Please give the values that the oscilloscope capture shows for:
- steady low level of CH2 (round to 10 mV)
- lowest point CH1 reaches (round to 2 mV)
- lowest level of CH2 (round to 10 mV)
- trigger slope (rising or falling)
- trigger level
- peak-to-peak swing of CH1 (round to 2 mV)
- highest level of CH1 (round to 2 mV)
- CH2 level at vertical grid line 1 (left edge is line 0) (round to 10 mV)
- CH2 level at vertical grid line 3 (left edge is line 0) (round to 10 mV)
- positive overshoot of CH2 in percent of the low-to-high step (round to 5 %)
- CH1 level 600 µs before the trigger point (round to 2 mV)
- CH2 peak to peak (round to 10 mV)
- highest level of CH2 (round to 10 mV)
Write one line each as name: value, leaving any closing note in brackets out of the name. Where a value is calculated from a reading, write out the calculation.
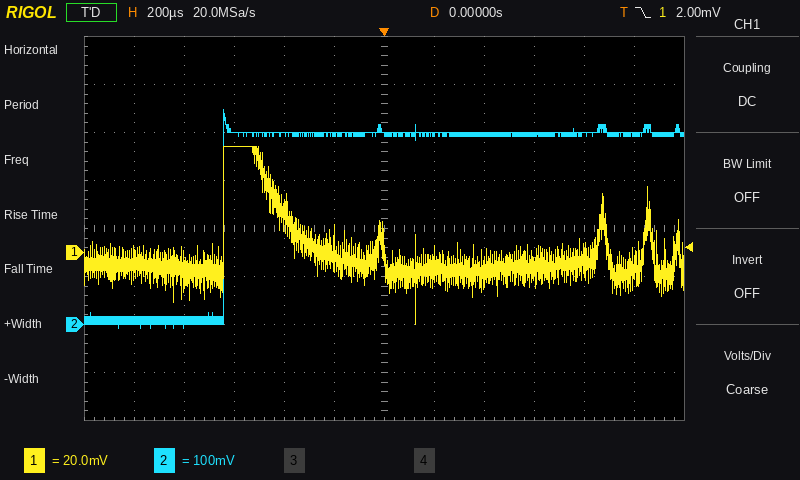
steady low level of CH2: 10 mV
lowest point CH1 reaches: -30 mV
lowest level of CH2: -10 mV
trigger slope: falling
trigger level: 2.00 mV
peak-to-peak swing of CH1: 44 mV − (-30 mV) = 74 mV
highest level of CH1: 44 mV
CH2 level at vertical grid line 1 (left edge is line 0): 10 mV
CH2 level at vertical grid line 3 (left edge is line 0): 400 mV
positive overshoot of CH2 in percent of the low-to-high step: 15 %
CH1 level 600 µs before the trigger point: 44 mV
CH2 peak to peak: 450 mV − (-10 mV) = 460 mV
highest level of CH2: 450 mV
